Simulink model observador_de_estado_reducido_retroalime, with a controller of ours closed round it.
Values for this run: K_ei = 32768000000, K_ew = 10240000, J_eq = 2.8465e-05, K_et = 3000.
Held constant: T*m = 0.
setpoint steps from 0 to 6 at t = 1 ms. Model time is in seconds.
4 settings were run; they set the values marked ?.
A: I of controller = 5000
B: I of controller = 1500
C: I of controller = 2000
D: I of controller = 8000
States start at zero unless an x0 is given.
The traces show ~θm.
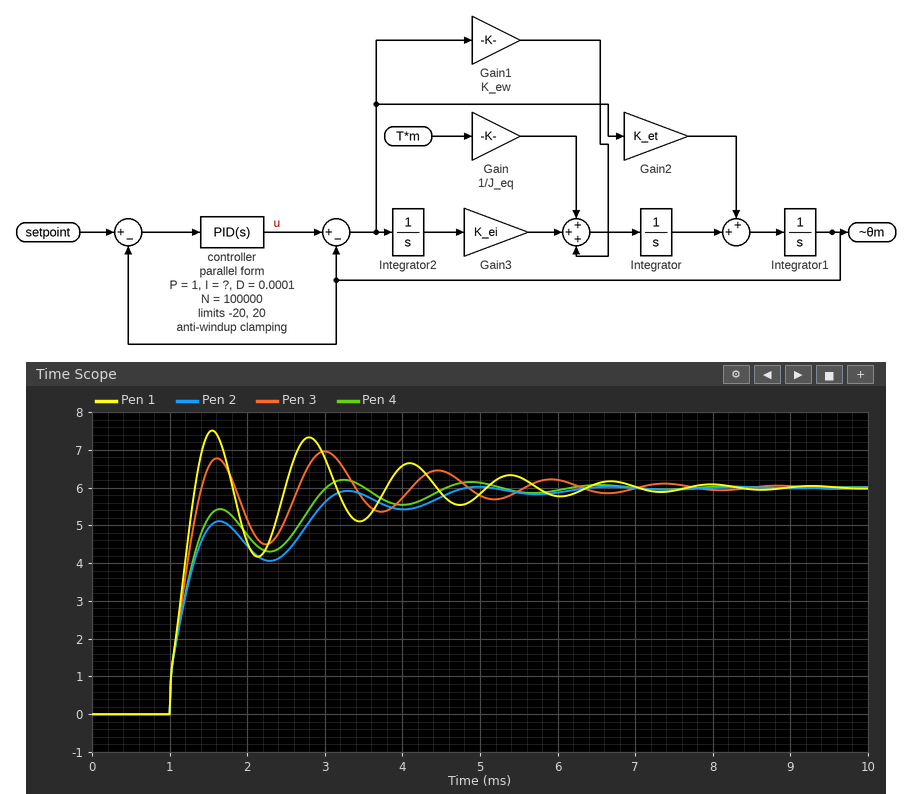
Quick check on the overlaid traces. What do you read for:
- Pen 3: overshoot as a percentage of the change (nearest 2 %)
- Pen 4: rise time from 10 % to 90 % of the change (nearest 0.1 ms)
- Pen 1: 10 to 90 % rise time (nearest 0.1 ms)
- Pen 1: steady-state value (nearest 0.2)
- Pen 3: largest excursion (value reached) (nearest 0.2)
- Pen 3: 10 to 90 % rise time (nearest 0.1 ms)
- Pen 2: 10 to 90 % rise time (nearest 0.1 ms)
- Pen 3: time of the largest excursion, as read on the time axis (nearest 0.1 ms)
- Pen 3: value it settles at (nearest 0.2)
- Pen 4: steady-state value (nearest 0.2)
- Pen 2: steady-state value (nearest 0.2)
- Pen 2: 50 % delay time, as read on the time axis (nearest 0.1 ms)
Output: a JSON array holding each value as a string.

["16 %", "0.6 ms", "0.3 ms", "6.0", "7.0", "0.3 ms", "1.9 ms", "3.0 ms", "6.0", "6.0", "6.0", "1.2 ms"]
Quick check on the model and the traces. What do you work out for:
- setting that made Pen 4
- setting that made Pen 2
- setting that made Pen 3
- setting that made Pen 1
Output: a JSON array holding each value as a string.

["C", "B", "A", "D"]
